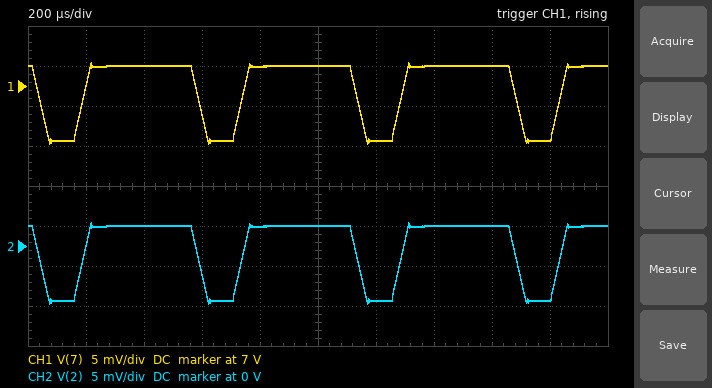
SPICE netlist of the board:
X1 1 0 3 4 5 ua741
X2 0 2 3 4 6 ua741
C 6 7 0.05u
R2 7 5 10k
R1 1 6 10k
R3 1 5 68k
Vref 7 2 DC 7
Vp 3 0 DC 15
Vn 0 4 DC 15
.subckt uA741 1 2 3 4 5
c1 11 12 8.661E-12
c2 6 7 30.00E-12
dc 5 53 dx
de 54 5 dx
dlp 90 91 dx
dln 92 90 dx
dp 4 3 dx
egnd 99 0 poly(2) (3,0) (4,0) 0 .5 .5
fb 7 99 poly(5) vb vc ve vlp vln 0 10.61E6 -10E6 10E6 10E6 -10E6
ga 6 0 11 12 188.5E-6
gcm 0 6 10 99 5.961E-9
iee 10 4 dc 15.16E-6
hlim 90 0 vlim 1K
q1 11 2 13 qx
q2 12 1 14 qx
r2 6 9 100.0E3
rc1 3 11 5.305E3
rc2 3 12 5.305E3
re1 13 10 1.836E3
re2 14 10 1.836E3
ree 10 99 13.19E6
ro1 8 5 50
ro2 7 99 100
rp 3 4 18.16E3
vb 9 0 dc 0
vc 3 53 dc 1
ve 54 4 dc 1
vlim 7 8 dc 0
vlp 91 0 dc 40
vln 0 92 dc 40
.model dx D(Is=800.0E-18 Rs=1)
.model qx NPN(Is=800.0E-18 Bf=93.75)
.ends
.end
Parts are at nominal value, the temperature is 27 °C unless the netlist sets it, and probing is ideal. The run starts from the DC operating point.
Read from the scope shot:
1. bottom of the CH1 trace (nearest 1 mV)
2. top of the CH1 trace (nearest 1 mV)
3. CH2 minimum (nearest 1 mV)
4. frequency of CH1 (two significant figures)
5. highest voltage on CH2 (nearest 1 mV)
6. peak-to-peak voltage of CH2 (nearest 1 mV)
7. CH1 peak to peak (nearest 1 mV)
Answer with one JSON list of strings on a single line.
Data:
["6.993 V", "7.003 V", "-7 mV", "1.8 kHz", "3 mV", "10 mV", "10 mV"]
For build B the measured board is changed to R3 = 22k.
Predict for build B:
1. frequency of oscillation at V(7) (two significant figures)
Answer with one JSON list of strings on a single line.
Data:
["740 Hz"]
